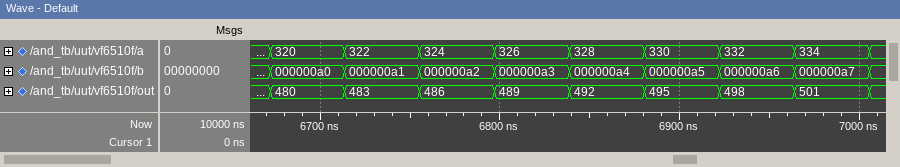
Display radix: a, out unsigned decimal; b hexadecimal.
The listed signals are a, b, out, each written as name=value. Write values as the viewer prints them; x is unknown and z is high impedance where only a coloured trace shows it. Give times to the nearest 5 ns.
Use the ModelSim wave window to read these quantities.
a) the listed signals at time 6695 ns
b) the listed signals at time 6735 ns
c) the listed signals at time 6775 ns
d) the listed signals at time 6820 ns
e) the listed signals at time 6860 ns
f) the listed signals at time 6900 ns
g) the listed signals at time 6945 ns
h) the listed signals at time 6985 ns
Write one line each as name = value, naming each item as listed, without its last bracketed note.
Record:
the listed signals at time 6695 ns = a=320, b=000000a0, out=480
the listed signals at time 6735 ns = a=322, b=000000a1, out=483
the listed signals at time 6775 ns = a=324, b=000000a2, out=486
the listed signals at time 6820 ns = a=326, b=000000a3, out=489
the listed signals at time 6860 ns = a=328, b=000000a4, out=492
the listed signals at time 6900 ns = a=330, b=000000a5, out=495
the listed signals at time 6945 ns = a=332, b=000000a6, out=498
the listed signals at time 6985 ns = a=334, b=000000a7, out=501
